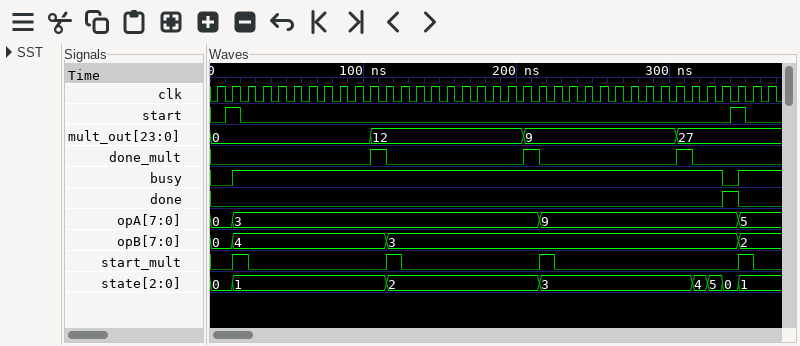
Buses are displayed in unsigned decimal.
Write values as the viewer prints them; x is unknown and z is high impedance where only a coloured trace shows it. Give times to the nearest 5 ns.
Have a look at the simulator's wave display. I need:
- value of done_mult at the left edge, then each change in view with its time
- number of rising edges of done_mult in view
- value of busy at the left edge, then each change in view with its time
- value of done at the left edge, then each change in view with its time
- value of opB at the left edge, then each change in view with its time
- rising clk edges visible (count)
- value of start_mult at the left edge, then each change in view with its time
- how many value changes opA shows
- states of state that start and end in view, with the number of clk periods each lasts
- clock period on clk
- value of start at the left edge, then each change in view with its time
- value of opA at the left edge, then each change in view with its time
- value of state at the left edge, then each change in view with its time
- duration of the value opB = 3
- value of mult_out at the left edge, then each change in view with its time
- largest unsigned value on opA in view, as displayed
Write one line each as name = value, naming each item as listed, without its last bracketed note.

value of done_mult at the left edge, then each change in view with its time = 0, 1 at 105 ns, 0 at 115 ns, 1 at 205 ns, 0 at 215 ns, 1 at 305 ns, 0 at 315 ns
number of rising edges of done_mult in view = 3
value of busy at the left edge, then each change in view with its time = 0, 1 at 15 ns, 0 at 335 ns, 1 at 345 ns
value of done at the left edge, then each change in view with its time = 0, 1 at 335 ns, 0 at 345 ns
value of opB at the left edge, then each change in view with its time = 0, 4 at 15 ns, 3 at 115 ns, 2 at 345 ns
rising clk edges visible = 37
value of start_mult at the left edge, then each change in view with its time = 0, 1 at 15 ns, 0 at 25 ns, 1 at 115 ns, 0 at 125 ns, 1 at 215 ns, 0 at 225 ns, 1 at 345 ns, 0 at 355 ns
how many value changes opA shows = 3
states of state that start and end in view, with the number of clk periods each lasts = 1: 10, 2: 10, 3: 10, 4: 1, 5: 1, 0: 1
clock period on clk = 10 ns
value of start at the left edge, then each change in view with its time = 0, 1 at 10 ns, 0 at 20 ns, 1 at 340 ns, 0 at 350 ns
value of opA at the left edge, then each change in view with its time = 0, 3 at 15 ns, 9 at 215 ns, 5 at 345 ns
value of state at the left edge, then each change in view with its time = 0, 1 at 15 ns, 2 at 115 ns, 3 at 215 ns, 4 at 315 ns, 5 at 325 ns, 0 at 335 ns, 1 at 345 ns
duration of the value opB = 3 = 230 ns
value of mult_out at the left edge, then each change in view with its time = 0, 12 at 105 ns, 9 at 205 ns, 27 at 305 ns
largest unsigned value on opA in view, as displayed = 9
